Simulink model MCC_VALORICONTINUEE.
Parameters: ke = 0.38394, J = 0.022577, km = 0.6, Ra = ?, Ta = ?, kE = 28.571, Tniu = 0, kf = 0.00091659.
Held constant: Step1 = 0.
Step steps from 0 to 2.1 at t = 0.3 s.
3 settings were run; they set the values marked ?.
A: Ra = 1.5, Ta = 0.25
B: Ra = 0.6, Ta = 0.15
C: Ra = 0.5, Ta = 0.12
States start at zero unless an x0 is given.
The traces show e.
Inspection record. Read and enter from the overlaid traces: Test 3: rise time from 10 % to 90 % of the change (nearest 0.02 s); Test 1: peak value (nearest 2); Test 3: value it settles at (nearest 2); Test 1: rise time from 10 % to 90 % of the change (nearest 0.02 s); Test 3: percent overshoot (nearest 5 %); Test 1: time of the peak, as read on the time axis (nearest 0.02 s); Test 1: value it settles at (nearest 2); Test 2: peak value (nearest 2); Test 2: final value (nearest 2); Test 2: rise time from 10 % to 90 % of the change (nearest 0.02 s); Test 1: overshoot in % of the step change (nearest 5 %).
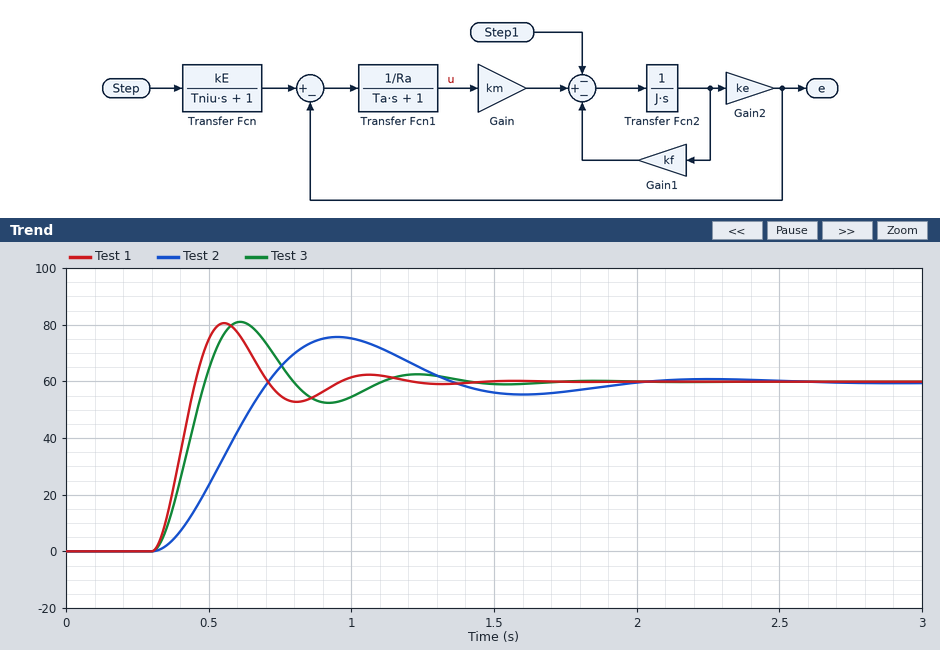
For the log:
0.12 s
80
60
0.10 s
35 %
0.56 s
60
76
60
0.28 s
35 %
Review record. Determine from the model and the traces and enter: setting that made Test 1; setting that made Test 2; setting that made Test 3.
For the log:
C
A
B
